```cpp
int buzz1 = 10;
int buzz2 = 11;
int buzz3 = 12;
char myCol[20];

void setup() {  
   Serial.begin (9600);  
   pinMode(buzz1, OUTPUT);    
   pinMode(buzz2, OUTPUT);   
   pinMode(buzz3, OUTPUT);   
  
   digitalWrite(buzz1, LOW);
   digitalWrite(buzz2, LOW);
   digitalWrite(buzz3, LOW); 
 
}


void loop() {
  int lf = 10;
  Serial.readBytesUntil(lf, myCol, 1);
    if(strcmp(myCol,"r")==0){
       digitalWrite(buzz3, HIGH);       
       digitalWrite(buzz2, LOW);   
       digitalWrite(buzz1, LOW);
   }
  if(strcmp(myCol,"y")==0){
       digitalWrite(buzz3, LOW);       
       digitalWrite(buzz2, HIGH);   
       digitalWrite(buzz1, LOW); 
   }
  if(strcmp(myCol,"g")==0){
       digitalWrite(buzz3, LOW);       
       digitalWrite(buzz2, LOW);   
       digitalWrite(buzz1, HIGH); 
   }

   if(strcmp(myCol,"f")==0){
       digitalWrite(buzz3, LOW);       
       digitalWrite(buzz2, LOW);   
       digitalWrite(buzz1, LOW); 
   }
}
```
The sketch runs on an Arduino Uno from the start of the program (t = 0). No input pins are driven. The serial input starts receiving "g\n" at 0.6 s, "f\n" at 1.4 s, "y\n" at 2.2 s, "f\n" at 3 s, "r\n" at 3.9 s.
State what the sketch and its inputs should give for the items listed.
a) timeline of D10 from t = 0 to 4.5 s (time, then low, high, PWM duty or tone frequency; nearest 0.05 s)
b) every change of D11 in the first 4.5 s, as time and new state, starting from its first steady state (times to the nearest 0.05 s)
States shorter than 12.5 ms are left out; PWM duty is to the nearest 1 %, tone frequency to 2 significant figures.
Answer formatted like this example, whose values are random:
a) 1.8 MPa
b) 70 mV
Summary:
a) 0 s low; 0.6 s high; 1.4 s low
b) 0 s low; 2.2 s high; 3 s low
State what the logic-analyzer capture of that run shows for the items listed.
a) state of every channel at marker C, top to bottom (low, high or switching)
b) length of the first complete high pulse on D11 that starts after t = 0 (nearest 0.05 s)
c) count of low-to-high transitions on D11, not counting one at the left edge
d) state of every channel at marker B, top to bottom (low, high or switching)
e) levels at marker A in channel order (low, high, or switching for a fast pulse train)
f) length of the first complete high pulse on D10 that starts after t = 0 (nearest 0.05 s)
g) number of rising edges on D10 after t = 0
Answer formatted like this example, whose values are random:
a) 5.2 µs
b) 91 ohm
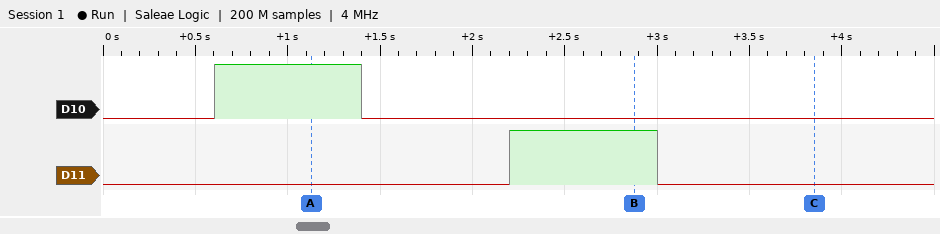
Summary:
a) D10 low, D11 low
b) 0.80 s
c) 1
d) D10 low, D11 high
e) D10 high, D11 low
f) 0.80 s
g) 1
